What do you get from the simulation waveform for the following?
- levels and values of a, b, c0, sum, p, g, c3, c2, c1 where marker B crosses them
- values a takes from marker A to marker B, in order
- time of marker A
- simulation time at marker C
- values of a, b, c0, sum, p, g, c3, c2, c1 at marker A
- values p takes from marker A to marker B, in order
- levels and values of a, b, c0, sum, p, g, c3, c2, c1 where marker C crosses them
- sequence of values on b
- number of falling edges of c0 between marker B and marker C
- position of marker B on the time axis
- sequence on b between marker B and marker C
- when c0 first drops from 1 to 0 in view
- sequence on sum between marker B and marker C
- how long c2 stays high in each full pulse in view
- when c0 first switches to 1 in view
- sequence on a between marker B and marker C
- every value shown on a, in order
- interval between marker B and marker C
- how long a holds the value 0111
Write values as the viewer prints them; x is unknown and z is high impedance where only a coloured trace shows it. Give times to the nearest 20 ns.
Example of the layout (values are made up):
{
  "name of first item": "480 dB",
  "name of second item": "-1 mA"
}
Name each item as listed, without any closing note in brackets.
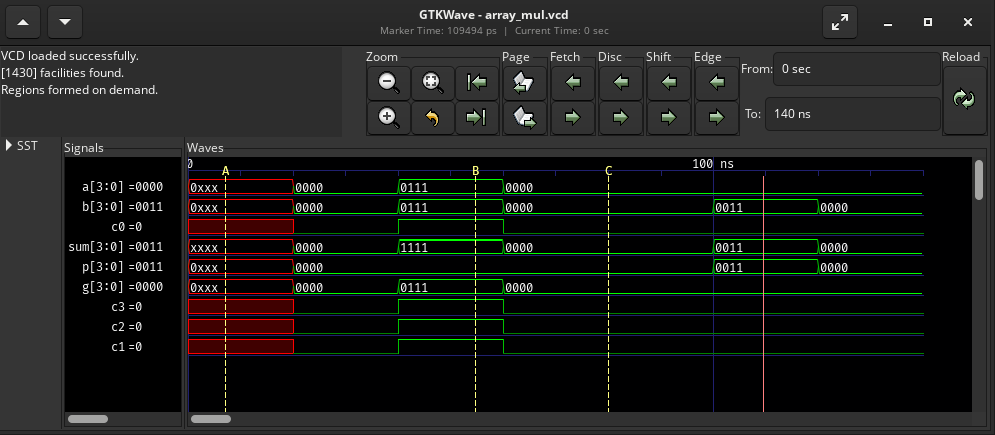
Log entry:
{
  "levels and values of a, b, c0, sum, p, g, c3, c2, c1 where marker B crosses them": "a=0111, b=0111, c0=1, sum=1111, p=0000, g=0111, c3=1, c2=1, c1=1",
  "values a takes from marker A to marker B, in order": "0xxx, 0000, 0111",
  "time of marker A": "0 ns",
  "simulation time at marker C": "80 ns",
  "values of a, b, c0, sum, p, g, c3, c2, c1 at marker A": "a=0xxx, b=0xxx, c0=x, sum=xxxx, p=0xxx, g=0xxx, c3=x, c2=x, c1=x",
  "values p takes from marker A to marker B, in order": "0xxx, 0000",
  "levels and values of a, b, c0, sum, p, g, c3, c2, c1 where marker C crosses them": "a=0000, b=0000, c0=0, sum=0000, p=0000, g=0000, c3=0, c2=0, c1=0",
  "sequence of values on b": "0xxx, 0000, 0111, 0000, 0011, 0000",
  "number of falling edges of c0 between marker B and marker C": "1",
  "position of marker B on the time axis": "60 ns",
  "sequence on b between marker B and marker C": "0111, 0000",
  "when c0 first drops from 1 to 0 in view": "60 ns",
  "sequence on sum between marker B and marker C": "1111, 0000",
  "how long c2 stays high in each full pulse in view": "20 ns",
  "when c0 first switches to 1 in view": "40 ns",
  "sequence on a between marker B and marker C": "0111, 0000",
  "every value shown on a, in order": "0xxx, 0000, 0111, 0000",
  "interval between marker B and marker C": "20 ns",
  "how long a holds the value 0111": "20 ns"
}
